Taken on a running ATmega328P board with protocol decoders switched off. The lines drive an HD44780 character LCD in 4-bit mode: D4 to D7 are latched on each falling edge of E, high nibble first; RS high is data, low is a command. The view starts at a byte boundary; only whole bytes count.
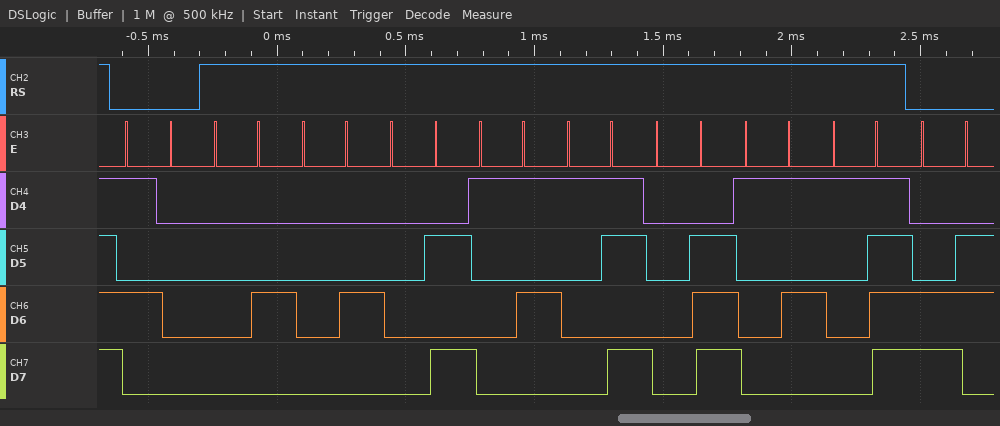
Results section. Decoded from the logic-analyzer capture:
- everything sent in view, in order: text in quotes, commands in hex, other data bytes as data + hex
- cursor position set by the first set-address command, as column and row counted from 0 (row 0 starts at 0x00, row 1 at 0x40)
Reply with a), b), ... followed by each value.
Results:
a) 0x50 data 04 04 0A 15 1B 0E 15 1F 0xC6
b) column 6, row 1
